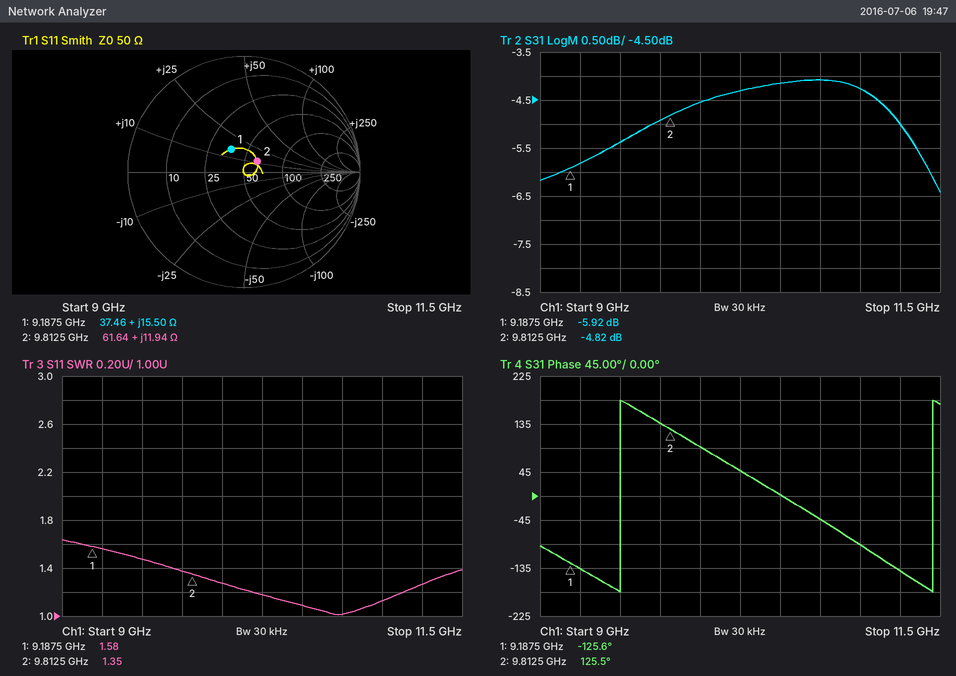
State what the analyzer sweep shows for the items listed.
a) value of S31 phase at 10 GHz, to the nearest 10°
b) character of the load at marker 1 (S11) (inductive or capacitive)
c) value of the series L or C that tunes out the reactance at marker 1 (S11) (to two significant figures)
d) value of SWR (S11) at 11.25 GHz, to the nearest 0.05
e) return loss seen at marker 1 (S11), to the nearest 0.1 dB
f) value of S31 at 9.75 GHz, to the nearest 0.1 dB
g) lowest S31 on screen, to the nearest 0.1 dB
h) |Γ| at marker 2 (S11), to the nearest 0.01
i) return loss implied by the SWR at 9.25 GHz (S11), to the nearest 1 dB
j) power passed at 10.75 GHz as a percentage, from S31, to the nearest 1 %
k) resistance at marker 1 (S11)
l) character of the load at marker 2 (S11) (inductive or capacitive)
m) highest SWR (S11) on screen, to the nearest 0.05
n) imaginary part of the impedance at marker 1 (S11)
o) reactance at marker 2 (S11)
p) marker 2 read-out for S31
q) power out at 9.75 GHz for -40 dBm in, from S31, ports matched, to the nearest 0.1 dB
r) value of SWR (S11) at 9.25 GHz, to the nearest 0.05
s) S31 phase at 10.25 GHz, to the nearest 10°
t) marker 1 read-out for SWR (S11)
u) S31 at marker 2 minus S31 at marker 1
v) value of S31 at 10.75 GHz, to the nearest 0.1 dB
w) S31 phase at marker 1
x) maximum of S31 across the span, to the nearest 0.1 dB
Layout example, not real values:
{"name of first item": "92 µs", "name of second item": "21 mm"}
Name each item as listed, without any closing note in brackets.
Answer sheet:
{"value of S31 phase at 10 GHz, to the nearest 10°": "90°", "character of the load at marker 1 (S11)": "inductive", "value of the series L or C that tunes out the reactance at marker 1 (S11)": "1.1 pF", "value of SWR (S11) at 11.25 GHz, to the nearest 0.05": "1.25", "return loss seen at marker 1 (S11), to the nearest 0.1 dB": "13.0 dB", "value of S31 at 9.75 GHz, to the nearest 0.1 dB": "-4.9 dB", "lowest S31 on screen, to the nearest 0.1 dB": "-6.4 dB", "|Γ| at marker 2 (S11), to the nearest 0.01": "0.15", "return loss implied by the SWR at 9.25 GHz (S11), to the nearest 1 dB": "13 dB", "power passed at 10.75 GHz as a percentage, from S31, to the nearest 1 %": "39 %", "resistance at marker 1": "37.46 Ω", "character of the load at marker 2 (S11)": "inductive", "highest SWR (S11) on screen, to the nearest 0.05": "1.65", "imaginary part of the impedance at marker 1": "+15.50 Ω", "reactance at marker 2": "+11.94 Ω", "marker 2 read-out for S31": "-4.82 dB", "power out at 9.75 GHz for -40 dBm in, from S31, ports matched, to the nearest 0.1 dB": "-44.9 dBm", "value of SWR (S11) at 9.25 GHz, to the nearest 0.05": "1.55", "S31 phase at 10.25 GHz, to the nearest 10°": "50°", "marker 1 read-out for SWR": "1.58", "S31 at marker 2 minus S31 at marker 1": "1.10 dB", "value of S31 at 10.75 GHz, to the nearest 0.1 dB": "-4.1 dB", "S31 phase at marker 1": "-125.6°", "maximum of S31 across the span, to the nearest 0.1 dB": "-4.1 dB"}
